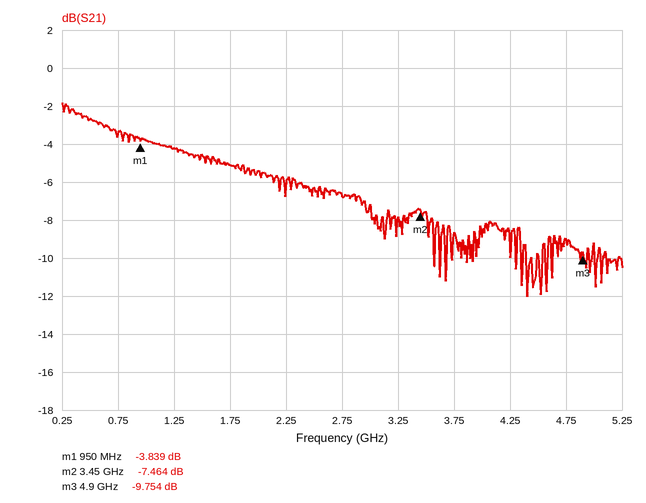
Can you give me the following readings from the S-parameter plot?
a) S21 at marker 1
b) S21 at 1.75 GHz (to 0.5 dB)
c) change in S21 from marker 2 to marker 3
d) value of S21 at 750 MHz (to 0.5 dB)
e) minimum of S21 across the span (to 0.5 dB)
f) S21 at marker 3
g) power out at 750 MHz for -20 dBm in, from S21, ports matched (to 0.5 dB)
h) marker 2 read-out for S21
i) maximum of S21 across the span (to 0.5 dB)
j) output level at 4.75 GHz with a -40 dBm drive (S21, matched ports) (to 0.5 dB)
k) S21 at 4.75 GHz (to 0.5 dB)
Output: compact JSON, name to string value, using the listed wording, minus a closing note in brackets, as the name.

{"S21 at marker 1": "-3.839 dB", "S21 at 1.75 GHz": "-5.0 dB", "change in S21 from marker 2 to marker 3": "-2.290 dB", "value of S21 at 750 MHz": "-3.5 dB", "minimum of S21 across the span": "-12.0 dB", "S21 at marker 3": "-9.754 dB", "power out at 750 MHz for -20 dBm in, from S21, ports matched": "-23.5 dBm", "marker 2 read-out for S21": "-7.464 dB", "maximum of S21 across the span": "-2.0 dB", "output level at 4.75 GHz with a -40 dBm drive (S21, matched ports)": "-49.0 dBm", "S21 at 4.75 GHz": "-9.0 dB"}
